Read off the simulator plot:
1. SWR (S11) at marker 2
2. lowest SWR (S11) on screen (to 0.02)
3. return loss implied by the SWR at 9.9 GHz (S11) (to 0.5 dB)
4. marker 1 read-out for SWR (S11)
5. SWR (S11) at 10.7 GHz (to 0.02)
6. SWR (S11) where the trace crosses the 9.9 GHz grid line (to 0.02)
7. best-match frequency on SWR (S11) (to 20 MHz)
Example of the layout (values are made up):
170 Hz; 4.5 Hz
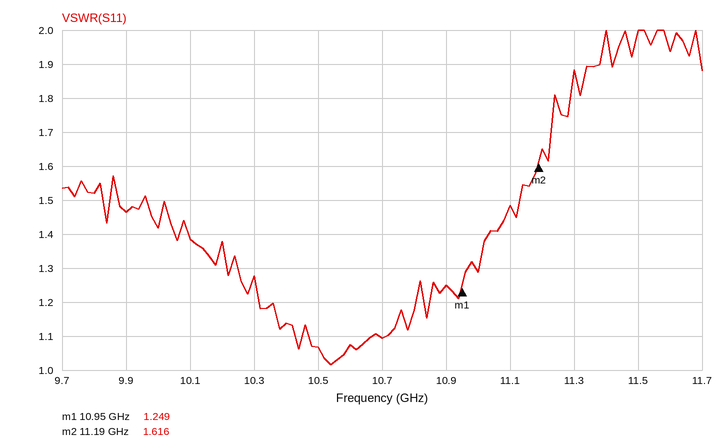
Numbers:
1.616; 1.02; 14.5 dB; 1.249; 1.10; 1.46; 10.54 GHz
